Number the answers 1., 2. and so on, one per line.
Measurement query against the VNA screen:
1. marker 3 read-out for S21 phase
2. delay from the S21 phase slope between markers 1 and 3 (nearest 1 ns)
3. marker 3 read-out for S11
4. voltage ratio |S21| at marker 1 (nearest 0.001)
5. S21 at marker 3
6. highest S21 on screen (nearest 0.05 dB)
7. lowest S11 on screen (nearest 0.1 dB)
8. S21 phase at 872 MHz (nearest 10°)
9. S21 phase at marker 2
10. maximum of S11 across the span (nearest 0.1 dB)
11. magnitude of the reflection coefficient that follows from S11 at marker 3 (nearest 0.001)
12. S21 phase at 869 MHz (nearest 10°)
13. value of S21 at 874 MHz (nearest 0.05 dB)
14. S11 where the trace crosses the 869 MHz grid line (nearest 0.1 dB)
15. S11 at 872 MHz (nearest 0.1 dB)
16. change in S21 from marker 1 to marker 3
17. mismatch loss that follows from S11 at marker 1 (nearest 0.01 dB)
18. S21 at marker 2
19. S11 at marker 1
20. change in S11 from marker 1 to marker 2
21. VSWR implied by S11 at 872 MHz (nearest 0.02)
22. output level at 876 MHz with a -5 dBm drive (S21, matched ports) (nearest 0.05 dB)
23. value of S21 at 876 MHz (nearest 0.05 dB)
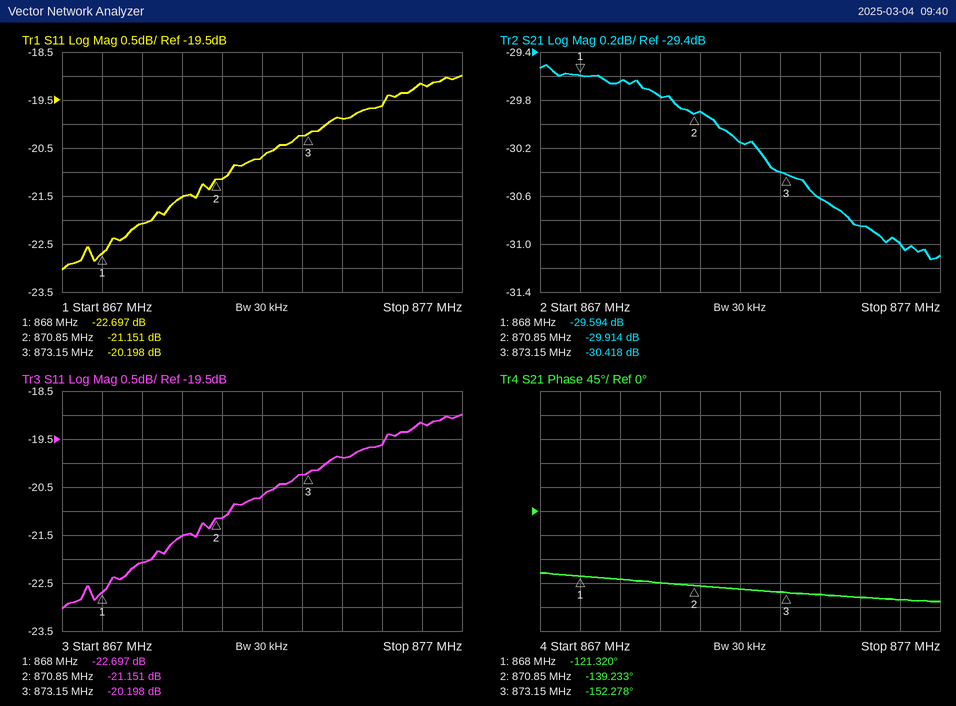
1. -152.278°
2. 17 ns
3. -20.198 dB
4. 0.033
5. -30.418 dB
6. -29.50 dB
7. -23.0 dB
8. -150°
9. -139.233°
10. -19.0 dB
11. 0.098
12. -130°
13. -30.60 dB
14. -22.1 dB
15. -20.7 dB
16. -0.824 dB
17. 0.02 dB
18. -29.914 dB
19. -22.697 dB
20. 1.546 dB
21. 1.20
22. -36.00 dBm
23. -31.00 dB
